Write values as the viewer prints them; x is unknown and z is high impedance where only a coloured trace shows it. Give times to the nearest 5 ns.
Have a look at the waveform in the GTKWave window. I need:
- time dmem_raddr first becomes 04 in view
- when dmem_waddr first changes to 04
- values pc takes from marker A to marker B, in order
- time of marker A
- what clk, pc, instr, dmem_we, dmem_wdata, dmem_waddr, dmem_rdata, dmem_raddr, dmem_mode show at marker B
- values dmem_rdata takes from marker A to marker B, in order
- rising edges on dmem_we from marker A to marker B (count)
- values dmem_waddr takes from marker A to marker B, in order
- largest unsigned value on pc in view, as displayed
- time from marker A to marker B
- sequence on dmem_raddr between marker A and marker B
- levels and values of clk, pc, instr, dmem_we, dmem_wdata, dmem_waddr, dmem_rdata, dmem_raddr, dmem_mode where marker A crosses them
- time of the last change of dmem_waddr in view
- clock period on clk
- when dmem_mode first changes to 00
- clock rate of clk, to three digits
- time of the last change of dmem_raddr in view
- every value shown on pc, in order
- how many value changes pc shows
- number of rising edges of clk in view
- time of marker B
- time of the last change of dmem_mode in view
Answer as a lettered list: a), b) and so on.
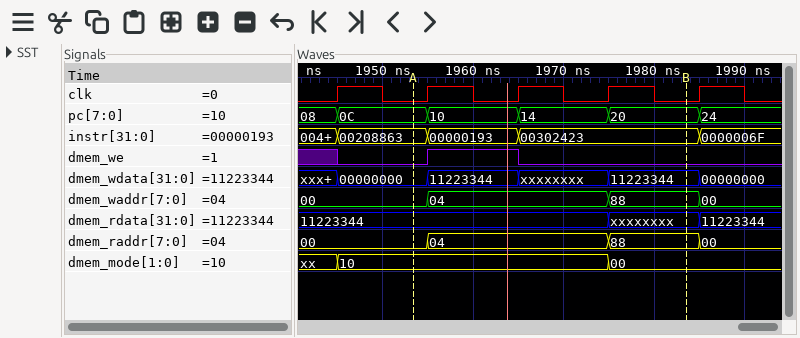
a) 1955 ns
b) 1955 ns
c) 0C, 10, 14, 20
d) 1955 ns
e) clk=0, pc=20, instr=00302423, dmem_we=0, dmem_wdata=11223344, dmem_waddr=88, dmem_rdata=xxxxxxxx, dmem_raddr=88, dmem_mode=00
f) 11223344, xxxxxxxx
g) 1
h) 00, 04, 88
i) 24
j) 30 ns
k) 00, 04, 88
l) clk=0, pc=0C, instr=00208863, dmem_we=0, dmem_wdata=00000000, dmem_waddr=00, dmem_rdata=11223344, dmem_raddr=00, dmem_mode=10
m) 1985 ns
n) 10 ns
o) 1975 ns
p) 100 MHz
q) 1985 ns
r) 08, 0C, 10, 14, 20, 24
s) 5
t) 5
u) 1985 ns
v) 1975 ns
